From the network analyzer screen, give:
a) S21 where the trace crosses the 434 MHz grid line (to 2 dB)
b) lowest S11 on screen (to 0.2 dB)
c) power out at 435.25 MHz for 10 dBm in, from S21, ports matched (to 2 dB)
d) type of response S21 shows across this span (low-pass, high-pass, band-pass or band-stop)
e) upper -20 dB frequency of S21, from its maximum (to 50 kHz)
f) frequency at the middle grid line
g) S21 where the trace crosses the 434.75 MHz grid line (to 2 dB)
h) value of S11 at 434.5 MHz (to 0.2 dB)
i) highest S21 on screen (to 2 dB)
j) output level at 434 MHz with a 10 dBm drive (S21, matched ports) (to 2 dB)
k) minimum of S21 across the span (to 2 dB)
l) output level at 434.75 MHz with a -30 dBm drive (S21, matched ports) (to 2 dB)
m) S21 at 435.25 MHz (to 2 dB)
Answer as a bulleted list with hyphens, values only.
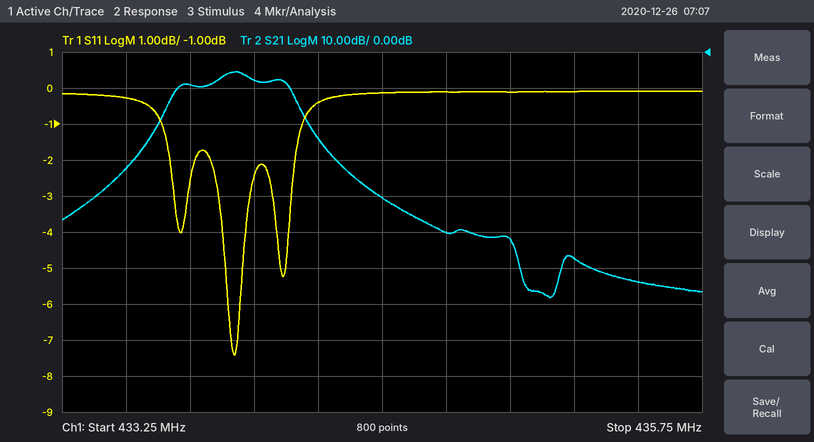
- -8 dB
- -7.4 dB
- -48 dBm
- band-pass
- 434.25 MHz
- 434.5 MHz
- -50 dB
- -0.2 dB
- -6 dB
- 2 dBm
- -68 dB
- -80 dBm
- -58 dB
